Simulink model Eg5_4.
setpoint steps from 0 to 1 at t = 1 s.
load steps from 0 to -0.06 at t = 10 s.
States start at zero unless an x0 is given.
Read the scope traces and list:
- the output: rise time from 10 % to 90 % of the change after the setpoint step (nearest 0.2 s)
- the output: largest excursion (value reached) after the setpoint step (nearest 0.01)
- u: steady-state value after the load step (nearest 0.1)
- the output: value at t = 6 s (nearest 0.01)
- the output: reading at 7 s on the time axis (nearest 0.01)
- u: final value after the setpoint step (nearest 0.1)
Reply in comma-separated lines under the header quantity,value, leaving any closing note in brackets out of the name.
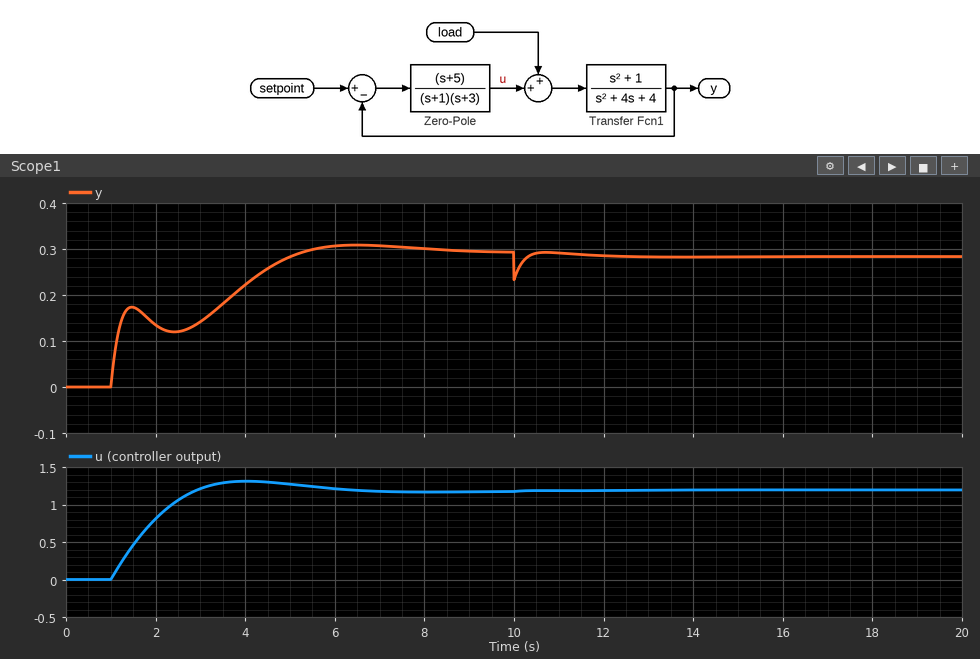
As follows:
quantity,value
the output: rise time from 10 % to 90 % of the change after the setpoint step,3.6 s
the output: largest excursion (value reached) after the setpoint step,0.31
u: steady-state value after the load step,1.2
the output: value at t = 6 s,0.31
the output: reading at 7 s on the time axis,0.31
u: final value after the setpoint step,1.2
